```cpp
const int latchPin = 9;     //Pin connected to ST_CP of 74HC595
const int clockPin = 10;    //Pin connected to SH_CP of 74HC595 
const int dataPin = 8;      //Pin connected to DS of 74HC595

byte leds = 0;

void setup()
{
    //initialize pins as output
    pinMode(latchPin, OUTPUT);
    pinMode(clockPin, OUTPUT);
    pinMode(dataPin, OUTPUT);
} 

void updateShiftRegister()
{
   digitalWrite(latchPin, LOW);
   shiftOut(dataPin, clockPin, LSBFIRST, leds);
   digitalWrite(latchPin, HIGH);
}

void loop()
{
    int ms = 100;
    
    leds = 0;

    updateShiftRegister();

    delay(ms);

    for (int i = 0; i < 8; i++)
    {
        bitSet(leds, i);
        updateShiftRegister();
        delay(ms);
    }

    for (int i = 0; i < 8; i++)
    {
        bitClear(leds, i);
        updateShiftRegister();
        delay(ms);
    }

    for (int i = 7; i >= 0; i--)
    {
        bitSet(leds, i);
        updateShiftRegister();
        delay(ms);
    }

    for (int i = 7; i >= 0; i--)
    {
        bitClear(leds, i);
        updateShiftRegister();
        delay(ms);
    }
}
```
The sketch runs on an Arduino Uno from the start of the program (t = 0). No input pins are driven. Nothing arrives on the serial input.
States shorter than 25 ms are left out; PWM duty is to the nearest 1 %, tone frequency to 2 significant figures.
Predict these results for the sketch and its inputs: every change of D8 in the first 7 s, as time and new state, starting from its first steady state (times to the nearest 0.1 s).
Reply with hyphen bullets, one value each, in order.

- 0 s low; 0.8 s high; 1.6 s low; 1.7 s high; 2.5 s low; 4.1 s high; 4.9 s low; 5 s high; 5.8 s low
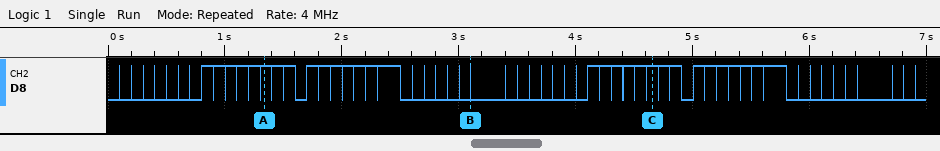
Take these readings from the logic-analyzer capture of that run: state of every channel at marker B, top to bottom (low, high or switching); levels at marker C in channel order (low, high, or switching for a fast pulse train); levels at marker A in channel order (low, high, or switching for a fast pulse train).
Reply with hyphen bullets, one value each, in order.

- D8 low
- D8 high
- D8 high
